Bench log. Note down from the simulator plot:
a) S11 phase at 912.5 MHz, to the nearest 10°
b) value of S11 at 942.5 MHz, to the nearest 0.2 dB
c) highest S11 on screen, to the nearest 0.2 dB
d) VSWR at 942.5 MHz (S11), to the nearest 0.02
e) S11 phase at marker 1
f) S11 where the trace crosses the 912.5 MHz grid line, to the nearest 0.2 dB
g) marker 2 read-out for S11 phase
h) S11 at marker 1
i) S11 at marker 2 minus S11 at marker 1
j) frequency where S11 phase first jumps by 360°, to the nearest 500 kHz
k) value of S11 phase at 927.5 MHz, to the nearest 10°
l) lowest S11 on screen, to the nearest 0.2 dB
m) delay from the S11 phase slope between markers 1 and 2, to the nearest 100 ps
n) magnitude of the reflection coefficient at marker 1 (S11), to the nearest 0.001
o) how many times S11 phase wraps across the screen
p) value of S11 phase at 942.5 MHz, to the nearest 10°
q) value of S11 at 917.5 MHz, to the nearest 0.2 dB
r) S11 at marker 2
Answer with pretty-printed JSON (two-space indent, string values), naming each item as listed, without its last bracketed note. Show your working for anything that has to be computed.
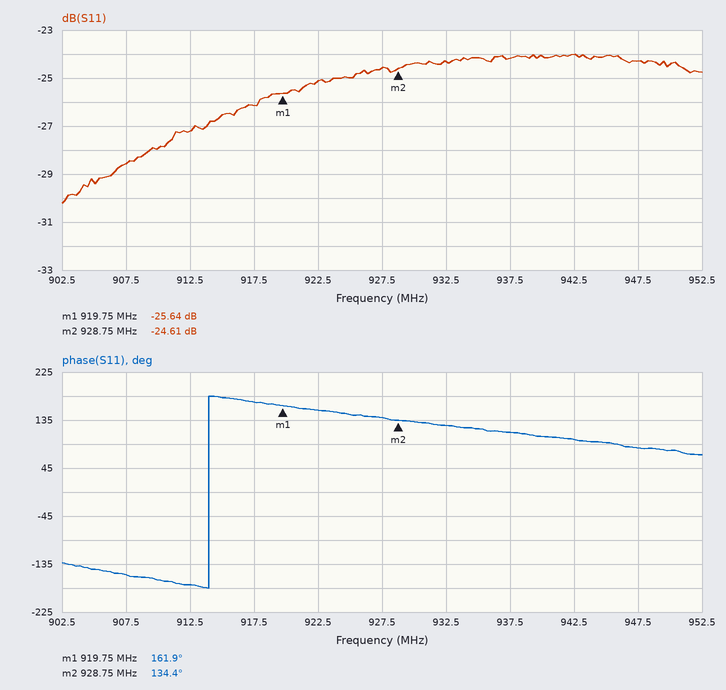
{
  "S11 phase at 912.5 MHz, to the nearest 10°": "-170°",
  "value of S11 at 942.5 MHz, to the nearest 0.2 dB": "-24.0 dB",
  "highest S11 on screen, to the nearest 0.2 dB": "-24.0 dB",
  "VSWR at 942.5 MHz (S11), to the nearest 0.02": "|Γ| = 10^(-24/20) = 0.0631; VSWR = (1 + 0.0631)/(1 − 0.0631) ≈ 1.13, so 1.14 to the nearest 0.02",
  "S11 phase at marker 1": "161.9°",
  "S11 where the trace crosses the 912.5 MHz grid line, to the nearest 0.2 dB": "-27.2 dB",
  "marker 2 read-out for S11 phase": "134.4°",
  "S11 at marker 1": "-25.64 dB",
  "S11 at marker 2 minus S11 at marker 1": "-24.61 − (-25.64) = 1.03 dB",
  "frequency where S11 phase first jumps by 360°, to the nearest 500 kHz": "914.0 MHz",
  "value of S11 phase at 927.5 MHz, to the nearest 10°": "140°",
  "lowest S11 on screen, to the nearest 0.2 dB": "-30.2 dB",
  "delay from the S11 phase slope between markers 1 and 2, to the nearest 100 ps": "−(134.4° − (161.9°))/(360° × 9 MHz) ≈ 8.5 ns",
  "magnitude of the reflection coefficient at marker 1 (S11), to the nearest 0.001": "10^(-25.64/20) ≈ 0.052",
  "how many times S11 phase wraps across the screen": "1",
  "value of S11 phase at 942.5 MHz, to the nearest 10°": "100°",
  "value of S11 at 917.5 MHz, to the nearest 0.2 dB": "-26.2 dB",
  "S11 at marker 2": "-24.61 dB"
}
